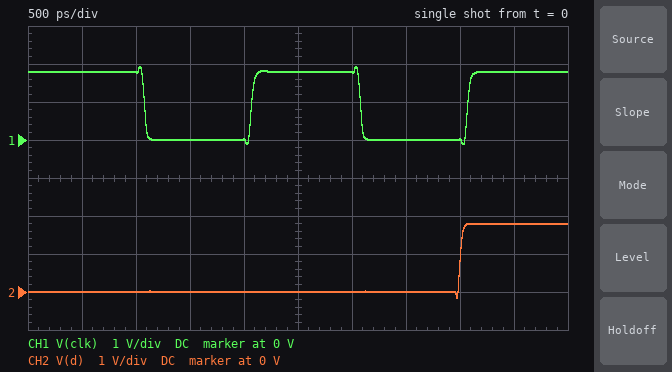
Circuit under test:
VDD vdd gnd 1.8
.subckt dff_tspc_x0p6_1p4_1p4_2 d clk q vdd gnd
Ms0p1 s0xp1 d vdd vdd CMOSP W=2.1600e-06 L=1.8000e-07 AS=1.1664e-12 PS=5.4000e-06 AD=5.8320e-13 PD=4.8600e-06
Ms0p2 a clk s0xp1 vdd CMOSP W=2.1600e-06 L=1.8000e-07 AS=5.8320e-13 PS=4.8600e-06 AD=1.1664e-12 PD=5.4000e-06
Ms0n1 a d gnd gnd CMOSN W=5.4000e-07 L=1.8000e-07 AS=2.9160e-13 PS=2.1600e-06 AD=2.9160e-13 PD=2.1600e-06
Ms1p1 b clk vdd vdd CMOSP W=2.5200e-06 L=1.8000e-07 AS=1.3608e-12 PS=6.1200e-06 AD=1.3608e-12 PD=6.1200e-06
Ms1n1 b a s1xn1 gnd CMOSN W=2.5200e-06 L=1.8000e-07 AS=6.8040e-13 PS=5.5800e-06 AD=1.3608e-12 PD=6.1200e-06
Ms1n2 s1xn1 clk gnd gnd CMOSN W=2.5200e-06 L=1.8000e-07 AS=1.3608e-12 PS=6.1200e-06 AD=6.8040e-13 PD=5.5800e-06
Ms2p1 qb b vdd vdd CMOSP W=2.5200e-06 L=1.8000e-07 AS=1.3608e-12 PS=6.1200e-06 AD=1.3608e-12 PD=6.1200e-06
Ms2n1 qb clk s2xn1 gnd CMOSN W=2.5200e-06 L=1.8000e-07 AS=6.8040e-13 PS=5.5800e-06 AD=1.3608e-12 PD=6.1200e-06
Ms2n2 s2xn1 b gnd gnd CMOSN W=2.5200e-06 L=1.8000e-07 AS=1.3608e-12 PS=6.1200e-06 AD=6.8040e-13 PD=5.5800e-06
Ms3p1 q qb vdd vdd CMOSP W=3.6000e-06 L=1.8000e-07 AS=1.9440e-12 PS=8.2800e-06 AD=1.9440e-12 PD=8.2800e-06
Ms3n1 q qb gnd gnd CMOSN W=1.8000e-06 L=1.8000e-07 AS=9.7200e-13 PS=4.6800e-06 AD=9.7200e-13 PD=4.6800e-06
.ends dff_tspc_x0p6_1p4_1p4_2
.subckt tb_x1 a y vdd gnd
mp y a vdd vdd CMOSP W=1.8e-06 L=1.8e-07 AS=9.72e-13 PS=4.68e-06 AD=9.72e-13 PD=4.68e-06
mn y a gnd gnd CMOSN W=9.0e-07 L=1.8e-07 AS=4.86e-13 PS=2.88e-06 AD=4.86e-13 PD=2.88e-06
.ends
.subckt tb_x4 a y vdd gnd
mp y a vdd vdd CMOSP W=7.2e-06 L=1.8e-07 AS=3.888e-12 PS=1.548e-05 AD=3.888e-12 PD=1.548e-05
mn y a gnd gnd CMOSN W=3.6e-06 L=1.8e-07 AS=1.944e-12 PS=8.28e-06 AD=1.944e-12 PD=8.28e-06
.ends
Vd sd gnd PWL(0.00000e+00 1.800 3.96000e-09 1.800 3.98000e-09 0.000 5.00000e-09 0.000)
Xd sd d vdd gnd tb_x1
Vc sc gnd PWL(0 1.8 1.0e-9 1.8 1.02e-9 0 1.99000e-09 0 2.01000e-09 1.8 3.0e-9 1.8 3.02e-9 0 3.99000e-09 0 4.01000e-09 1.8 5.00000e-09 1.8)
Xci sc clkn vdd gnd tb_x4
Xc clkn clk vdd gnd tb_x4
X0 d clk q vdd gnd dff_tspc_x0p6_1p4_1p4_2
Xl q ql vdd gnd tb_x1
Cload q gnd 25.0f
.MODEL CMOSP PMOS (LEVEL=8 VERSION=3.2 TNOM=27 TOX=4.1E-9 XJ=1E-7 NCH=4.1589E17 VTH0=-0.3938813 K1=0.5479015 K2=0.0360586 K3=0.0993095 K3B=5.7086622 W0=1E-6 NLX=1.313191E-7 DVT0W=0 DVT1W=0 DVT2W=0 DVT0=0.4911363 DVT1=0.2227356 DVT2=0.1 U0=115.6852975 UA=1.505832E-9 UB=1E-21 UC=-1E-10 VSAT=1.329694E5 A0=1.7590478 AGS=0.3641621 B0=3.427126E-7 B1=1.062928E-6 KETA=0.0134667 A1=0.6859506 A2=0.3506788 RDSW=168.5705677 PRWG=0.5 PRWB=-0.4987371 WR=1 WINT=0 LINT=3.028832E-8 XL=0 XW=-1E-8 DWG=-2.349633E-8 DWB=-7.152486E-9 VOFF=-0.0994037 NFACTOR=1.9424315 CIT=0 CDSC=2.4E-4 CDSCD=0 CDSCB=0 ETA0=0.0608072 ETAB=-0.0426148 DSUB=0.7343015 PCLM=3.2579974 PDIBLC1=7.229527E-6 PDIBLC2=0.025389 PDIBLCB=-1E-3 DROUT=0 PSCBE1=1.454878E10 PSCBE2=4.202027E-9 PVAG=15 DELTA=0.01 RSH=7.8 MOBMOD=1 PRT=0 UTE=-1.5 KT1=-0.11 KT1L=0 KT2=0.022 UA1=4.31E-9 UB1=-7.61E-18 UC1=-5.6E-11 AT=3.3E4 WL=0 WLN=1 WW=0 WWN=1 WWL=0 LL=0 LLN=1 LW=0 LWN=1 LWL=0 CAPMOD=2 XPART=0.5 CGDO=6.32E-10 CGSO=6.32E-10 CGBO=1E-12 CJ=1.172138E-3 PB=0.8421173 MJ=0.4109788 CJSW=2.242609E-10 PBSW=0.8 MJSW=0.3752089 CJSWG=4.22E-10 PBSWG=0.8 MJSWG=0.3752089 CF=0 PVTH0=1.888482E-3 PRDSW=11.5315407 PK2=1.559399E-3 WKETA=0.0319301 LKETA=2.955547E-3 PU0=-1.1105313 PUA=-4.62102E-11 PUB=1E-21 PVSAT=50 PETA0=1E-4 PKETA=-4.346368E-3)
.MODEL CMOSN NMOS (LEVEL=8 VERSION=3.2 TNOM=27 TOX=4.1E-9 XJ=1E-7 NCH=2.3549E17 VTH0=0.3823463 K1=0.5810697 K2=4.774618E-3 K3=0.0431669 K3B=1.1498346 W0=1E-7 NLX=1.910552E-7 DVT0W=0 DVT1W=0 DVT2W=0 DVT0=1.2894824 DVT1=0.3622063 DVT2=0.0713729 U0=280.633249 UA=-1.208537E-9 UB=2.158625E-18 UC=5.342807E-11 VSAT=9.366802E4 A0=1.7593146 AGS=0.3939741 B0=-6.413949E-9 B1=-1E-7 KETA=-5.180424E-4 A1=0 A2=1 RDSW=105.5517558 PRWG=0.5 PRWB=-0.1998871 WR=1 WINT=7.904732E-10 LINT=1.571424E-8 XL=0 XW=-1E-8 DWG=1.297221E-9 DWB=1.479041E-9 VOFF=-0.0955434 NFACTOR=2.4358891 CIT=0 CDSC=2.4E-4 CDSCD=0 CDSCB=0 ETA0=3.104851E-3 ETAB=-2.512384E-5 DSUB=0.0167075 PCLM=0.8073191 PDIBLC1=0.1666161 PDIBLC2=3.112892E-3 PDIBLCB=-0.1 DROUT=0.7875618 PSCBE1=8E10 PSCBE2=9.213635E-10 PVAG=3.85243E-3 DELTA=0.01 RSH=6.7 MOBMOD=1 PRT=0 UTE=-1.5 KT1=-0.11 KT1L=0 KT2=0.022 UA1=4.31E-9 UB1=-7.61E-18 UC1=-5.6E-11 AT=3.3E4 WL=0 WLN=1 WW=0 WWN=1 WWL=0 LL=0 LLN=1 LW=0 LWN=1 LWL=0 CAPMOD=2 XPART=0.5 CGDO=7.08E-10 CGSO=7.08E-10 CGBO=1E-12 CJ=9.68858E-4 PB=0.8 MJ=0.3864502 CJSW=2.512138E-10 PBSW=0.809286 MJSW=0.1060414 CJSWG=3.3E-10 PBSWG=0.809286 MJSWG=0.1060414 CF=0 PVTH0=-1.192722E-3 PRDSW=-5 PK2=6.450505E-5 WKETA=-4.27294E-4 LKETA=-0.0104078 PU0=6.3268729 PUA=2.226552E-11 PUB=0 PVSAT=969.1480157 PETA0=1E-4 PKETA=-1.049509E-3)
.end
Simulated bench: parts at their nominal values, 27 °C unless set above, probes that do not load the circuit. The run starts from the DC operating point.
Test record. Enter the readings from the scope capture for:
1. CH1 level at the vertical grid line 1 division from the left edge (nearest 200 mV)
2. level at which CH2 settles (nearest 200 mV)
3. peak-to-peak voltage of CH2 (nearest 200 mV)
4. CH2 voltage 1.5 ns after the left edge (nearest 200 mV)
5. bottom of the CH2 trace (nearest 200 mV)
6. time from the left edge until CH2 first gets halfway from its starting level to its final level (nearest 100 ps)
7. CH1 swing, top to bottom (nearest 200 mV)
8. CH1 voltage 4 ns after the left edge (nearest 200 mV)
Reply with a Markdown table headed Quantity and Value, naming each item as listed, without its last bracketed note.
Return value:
| Quantity | Value |
|---|---|
| CH1 level at the vertical grid line 1 division from the left edge | 1.8 V |
| level at which CH2 settles | 1.8 V |
| peak-to-peak voltage of CH2 | 2.0 V |
| CH2 voltage 1.5 ns after the left edge | 0 V |
| bottom of the CH2 trace | -200 mV |
| time from the left edge until CH2 first gets halfway from its starting level to its final level | 4.0 ns |
| CH1 swing, top to bottom | 2.0 V |
| CH1 voltage 4 ns after the left edge | 0 V |
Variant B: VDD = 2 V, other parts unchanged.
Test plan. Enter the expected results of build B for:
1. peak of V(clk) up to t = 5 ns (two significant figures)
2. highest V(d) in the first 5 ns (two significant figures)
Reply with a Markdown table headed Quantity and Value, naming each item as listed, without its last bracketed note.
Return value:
| Quantity | Value |
|---|---|
| peak of V(clk) up to t = 5 ns | 2.1 V |
| highest V(d) in the first 5 ns | 2.0 V |
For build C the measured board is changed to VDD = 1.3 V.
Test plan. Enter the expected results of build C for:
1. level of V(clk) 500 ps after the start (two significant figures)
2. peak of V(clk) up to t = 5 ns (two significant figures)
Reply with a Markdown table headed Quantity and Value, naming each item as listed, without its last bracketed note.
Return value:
| Quantity | Value |
|---|---|
| level of V(clk) 500 ps after the start | 1.3 V |
| peak of V(clk) up to t = 5 ns | 1.4 V |
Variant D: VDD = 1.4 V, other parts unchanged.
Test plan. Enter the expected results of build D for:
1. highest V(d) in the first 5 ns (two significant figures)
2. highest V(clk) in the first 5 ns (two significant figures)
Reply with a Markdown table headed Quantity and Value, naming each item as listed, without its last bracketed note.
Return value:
| Quantity | Value |
|---|---|
| highest V(d) in the first 5 ns | 1.4 V |
| highest V(clk) in the first 5 ns | 1.5 V |
